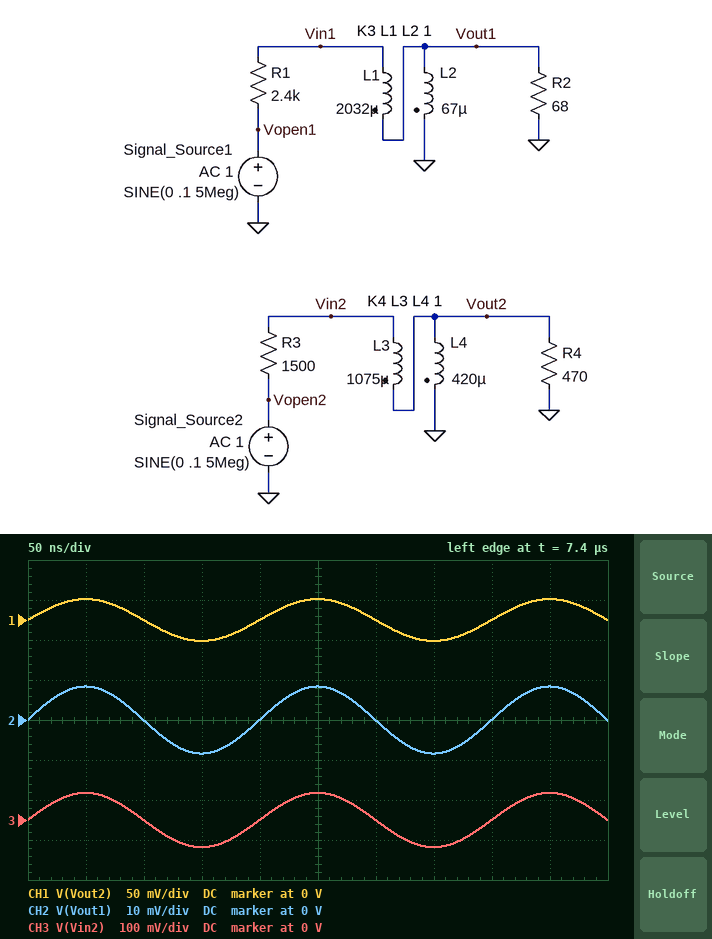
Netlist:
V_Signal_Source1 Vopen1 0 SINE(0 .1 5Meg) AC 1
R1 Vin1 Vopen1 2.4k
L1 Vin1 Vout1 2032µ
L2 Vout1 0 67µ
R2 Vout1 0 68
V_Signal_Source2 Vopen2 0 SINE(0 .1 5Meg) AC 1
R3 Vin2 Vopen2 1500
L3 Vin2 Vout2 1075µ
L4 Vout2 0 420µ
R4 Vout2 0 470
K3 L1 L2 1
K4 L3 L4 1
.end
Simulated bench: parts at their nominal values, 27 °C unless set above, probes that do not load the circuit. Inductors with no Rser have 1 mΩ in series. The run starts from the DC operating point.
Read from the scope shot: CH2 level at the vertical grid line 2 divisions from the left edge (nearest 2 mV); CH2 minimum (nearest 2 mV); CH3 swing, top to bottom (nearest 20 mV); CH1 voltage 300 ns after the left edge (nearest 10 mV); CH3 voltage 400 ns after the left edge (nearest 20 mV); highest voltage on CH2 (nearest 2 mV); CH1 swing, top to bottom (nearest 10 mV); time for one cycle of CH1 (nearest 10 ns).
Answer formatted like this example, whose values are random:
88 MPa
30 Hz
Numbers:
0 V
-8 mV
140 mV
0 V
0 V
8 mV
50 mV
200 ns
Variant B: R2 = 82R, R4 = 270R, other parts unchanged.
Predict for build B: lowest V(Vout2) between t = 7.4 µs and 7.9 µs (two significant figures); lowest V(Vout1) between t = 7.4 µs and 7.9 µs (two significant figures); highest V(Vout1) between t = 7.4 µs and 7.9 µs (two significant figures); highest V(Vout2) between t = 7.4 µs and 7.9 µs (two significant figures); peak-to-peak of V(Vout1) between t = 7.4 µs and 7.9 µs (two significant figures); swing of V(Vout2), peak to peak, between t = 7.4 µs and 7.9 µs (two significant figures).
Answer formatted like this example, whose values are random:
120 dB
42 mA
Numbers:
-21 mV
-9.1 mV
9.1 mV
21 mV
18 mV
42 mV
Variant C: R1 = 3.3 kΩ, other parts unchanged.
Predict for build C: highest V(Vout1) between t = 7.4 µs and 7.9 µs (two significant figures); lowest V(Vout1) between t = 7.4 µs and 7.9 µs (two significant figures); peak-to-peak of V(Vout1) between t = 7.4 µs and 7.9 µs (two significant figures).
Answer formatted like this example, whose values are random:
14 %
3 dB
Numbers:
7.2 mV
-7.2 mV
14 mV
